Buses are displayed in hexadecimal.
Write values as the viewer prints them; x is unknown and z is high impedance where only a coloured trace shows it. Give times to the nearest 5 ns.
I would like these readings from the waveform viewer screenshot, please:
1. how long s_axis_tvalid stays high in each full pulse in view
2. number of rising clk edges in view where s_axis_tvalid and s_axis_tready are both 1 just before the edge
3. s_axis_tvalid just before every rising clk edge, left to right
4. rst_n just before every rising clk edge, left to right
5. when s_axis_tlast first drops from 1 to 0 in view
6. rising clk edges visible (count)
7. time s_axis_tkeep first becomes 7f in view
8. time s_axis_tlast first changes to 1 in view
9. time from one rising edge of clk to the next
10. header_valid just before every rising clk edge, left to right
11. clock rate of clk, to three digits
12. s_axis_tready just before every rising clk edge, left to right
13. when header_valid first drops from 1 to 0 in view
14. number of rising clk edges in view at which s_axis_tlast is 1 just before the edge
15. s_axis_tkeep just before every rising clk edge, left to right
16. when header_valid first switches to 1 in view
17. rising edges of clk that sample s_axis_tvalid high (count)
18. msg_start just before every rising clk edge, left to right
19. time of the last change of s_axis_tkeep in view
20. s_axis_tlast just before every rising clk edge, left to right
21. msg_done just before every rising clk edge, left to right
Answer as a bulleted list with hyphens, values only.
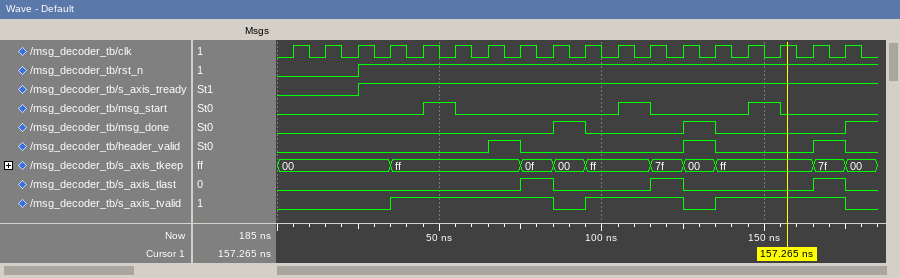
- 50 ns, 30 ns, 40 ns
- 12
- 0 0 0 0 1 1 1 1 1 0 1 1 1 0 1 1 1 1
- 0 0 0 1 1 1 1 1 1 1 1 1 1 1 1 1 1 1
- 85 ns
- 18
- 115 ns
- 75 ns
- 10 ns
- 0 0 0 0 0 0 0 1 0 0 0 0 0 1 0 0 0 1
- 100 MHz
- 0 0 0 1 1 1 1 1 1 1 1 1 1 1 1 1 1 1
- 75 ns
- 3
- 00, 00, 00, 00, ff, ff, ff, ff, 0f, 00, ff, ff, 7f, 00, ff, ff, ff, 7f
- 65 ns
- 12
- 0 0 0 0 0 1 0 0 0 0 0 1 0 0 0 1 0 0
- 175 ns
- 0 0 0 0 0 0 0 0 1 0 0 0 1 0 0 0 0 1
- 0 0 0 0 0 0 0 0 0 1 0 0 0 1 0 0 0 0
